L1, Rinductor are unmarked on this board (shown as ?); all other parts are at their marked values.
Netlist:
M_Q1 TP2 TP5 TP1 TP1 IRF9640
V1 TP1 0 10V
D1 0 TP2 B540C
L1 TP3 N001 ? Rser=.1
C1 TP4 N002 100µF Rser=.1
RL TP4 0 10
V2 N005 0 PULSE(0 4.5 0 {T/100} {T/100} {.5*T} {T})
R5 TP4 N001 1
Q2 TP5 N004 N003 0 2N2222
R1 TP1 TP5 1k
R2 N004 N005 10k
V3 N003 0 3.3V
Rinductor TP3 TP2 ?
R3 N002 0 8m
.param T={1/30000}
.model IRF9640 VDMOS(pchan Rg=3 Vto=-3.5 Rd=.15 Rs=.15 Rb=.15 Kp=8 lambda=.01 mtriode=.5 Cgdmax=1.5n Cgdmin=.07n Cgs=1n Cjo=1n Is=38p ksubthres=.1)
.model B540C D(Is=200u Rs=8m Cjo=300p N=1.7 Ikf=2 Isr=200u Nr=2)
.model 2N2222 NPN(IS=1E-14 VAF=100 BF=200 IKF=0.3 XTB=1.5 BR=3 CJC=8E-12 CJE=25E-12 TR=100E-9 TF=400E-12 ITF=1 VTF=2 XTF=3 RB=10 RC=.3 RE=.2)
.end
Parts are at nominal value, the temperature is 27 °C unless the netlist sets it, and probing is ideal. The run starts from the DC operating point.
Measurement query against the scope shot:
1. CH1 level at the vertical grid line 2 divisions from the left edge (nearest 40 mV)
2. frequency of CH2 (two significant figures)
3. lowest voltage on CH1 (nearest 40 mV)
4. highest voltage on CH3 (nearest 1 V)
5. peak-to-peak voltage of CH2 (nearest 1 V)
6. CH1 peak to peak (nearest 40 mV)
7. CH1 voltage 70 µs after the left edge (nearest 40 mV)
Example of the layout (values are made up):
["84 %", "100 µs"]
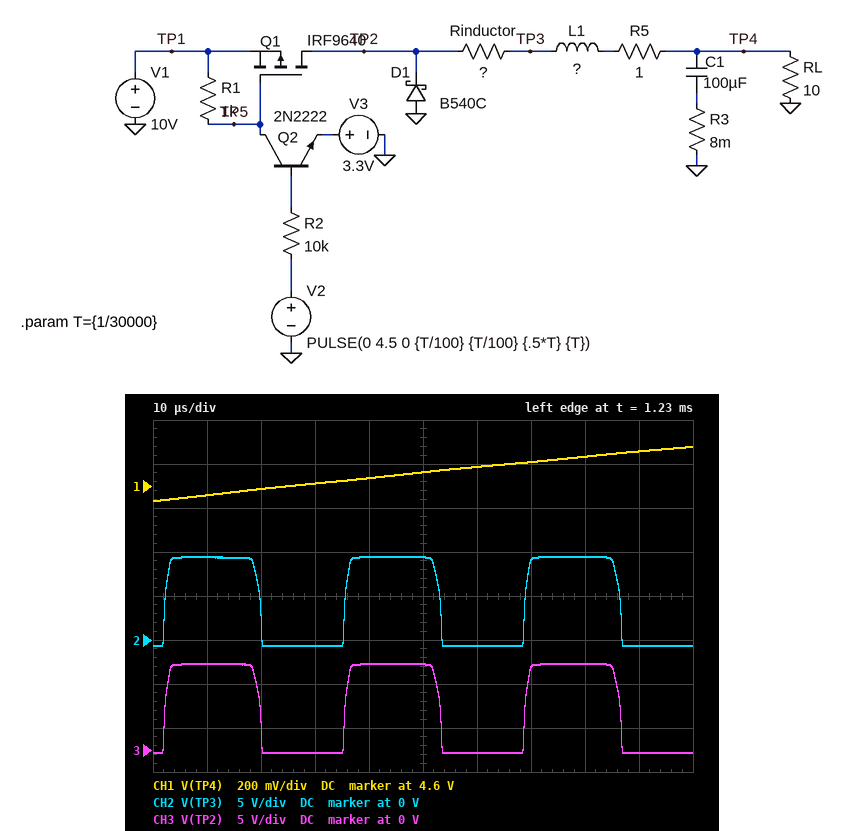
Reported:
["4.60 V", "30 kHz", "4.52 V", "10 V", "10 V", "240 mV", "4.72 V"]
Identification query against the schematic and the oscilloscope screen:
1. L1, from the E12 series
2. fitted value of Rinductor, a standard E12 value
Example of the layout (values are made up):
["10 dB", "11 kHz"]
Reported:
["3.3 mH", "0.47 Ω"]
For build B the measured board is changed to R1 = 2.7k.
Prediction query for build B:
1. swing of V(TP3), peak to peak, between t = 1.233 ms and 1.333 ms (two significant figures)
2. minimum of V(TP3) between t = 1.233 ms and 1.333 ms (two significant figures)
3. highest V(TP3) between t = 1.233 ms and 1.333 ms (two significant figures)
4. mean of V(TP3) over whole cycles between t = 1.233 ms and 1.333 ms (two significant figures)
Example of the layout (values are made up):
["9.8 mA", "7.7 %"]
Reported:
["10 V", "-830 mV", "9.2 V", "5.7 V"]
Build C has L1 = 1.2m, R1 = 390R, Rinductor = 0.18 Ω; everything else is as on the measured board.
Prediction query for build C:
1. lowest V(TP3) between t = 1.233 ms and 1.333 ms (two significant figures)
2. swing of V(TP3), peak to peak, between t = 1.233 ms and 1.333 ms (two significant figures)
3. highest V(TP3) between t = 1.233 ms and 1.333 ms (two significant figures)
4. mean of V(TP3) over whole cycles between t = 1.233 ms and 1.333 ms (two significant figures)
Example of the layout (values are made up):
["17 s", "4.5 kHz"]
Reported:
["-330 mV", "6.1 V", "5.8 V", "1.3 V"]
